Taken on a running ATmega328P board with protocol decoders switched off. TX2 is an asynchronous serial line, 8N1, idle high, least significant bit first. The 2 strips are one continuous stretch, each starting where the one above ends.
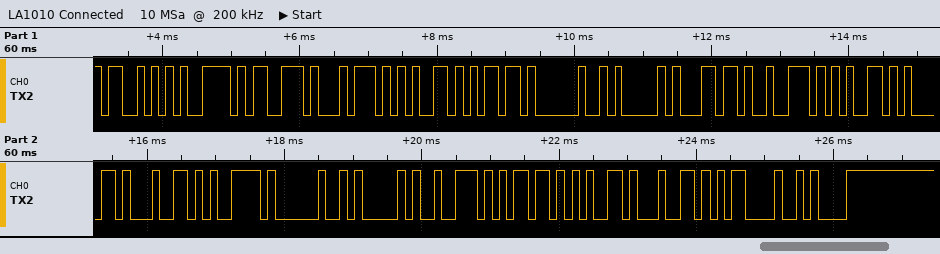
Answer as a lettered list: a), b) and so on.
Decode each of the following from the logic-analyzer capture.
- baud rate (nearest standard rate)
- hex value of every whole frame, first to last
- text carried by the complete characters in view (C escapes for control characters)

a) 9600 baud
b) 53 79 73 74 65 6D 20 41 6C 72 65 61 64 79 20 41 72 6D 65 64 0D 0A
c) "System Already Armed\r\n"
